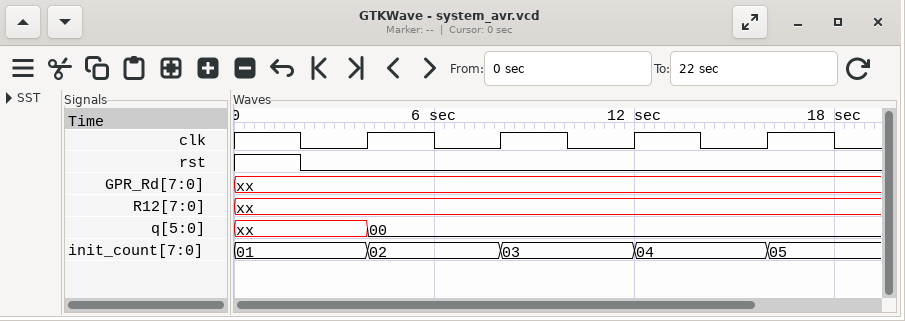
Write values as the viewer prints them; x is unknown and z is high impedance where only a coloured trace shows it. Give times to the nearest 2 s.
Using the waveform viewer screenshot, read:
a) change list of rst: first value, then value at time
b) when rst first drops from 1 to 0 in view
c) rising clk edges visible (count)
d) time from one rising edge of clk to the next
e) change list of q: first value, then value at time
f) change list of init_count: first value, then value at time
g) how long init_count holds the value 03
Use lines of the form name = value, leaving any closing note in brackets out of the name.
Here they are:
change list of rst: first value, then value at time = 1, 0 at 2 s
when rst first drops from 1 to 0 in view = 2 s
rising clk edges visible = 4
time from one rising edge of clk to the next = 4 s
change list of q: first value, then value at time = xx, 00 at 4 s
change list of init_count: first value, then value at time = 01, 02 at 4 s, 03 at 8 s, 04 at 12 s, 05 at 16 s
how long init_count holds the value 03 = 4 s
